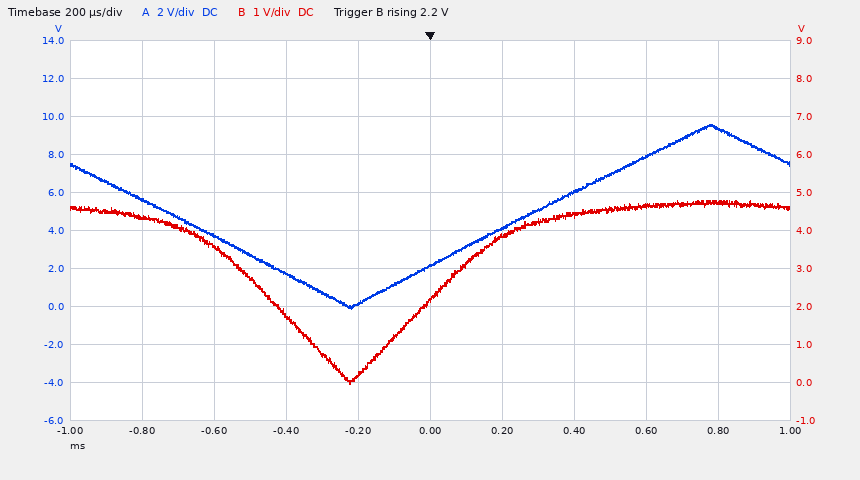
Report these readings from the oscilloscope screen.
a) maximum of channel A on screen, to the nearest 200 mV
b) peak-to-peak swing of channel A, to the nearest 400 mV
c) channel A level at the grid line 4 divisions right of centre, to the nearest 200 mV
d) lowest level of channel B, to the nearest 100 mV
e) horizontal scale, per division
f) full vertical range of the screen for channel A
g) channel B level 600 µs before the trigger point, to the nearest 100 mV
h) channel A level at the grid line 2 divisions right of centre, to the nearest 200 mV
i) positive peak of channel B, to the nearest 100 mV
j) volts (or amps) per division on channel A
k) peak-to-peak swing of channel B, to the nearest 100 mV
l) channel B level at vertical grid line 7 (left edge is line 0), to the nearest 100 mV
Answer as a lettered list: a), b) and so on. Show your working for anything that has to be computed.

a) 9.6 V
b) 9.6 V
c) 9.4 V
d) 0.0 V
e) 200 µs
f) 20 V
g) 3.6 V
h) 6.0 V
i) 4.8 V
j) 2 V
k) 4.8 V − (0.0 V) = 4.8 V
l) 4.4 V
